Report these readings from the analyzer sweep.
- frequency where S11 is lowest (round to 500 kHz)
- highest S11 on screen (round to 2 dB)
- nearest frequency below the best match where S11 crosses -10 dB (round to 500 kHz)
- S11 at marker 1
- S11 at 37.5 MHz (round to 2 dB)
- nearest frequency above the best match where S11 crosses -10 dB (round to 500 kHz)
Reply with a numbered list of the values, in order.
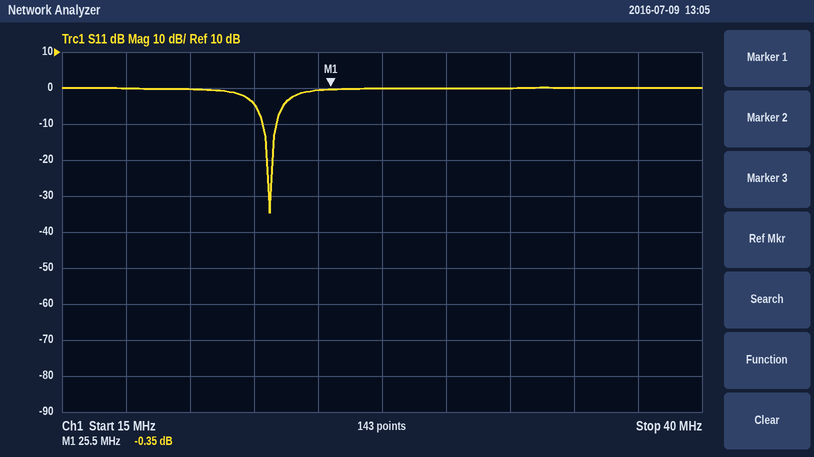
1. 23.0 MHz
2. 0 dB
3. 23.0 MHz
4. -0.35 dB
5. 0 dB
6. 23.5 MHz
